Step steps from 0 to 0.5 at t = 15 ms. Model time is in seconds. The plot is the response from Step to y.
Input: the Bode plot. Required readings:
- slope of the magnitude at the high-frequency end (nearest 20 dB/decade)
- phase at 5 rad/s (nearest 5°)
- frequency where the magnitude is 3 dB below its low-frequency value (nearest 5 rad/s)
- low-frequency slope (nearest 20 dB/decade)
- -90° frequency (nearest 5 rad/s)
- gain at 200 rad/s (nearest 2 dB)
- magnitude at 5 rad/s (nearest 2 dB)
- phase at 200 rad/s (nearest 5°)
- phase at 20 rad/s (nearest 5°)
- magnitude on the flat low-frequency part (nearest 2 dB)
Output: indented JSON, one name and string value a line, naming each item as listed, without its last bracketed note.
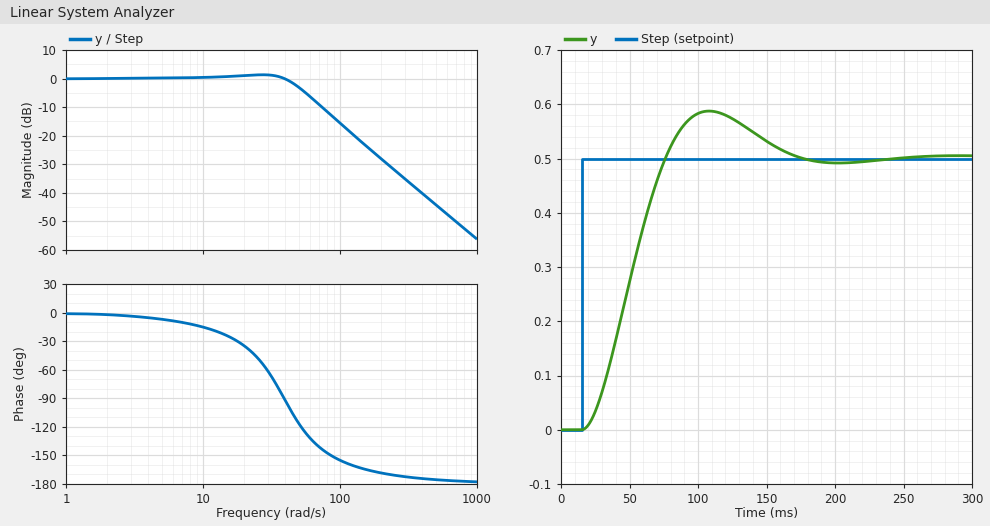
{
  "slope of the magnitude at the high-frequency end": "-40 dB/decade",
  "phase at 5 rad/s": "-5°",
  "frequency where the magnitude is 3 dB below its low-frequency value": "50 rad/s",
  "low-frequency slope": "0 dB/decade",
  "-90° frequency": "40 rad/s",
  "gain at 200 rad/s": "-28 dB",
  "magnitude at 5 rad/s": "0 dB",
  "phase at 200 rad/s": "-170°",
  "phase at 20 rad/s": "-35°",
  "magnitude on the flat low-frequency part": "0 dB"
}
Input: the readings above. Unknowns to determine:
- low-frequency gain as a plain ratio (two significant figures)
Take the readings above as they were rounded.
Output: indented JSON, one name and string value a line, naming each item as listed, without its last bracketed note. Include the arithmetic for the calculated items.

{
  "low-frequency gain as a plain ratio": "10^(0 / 20) = 1.0"
}
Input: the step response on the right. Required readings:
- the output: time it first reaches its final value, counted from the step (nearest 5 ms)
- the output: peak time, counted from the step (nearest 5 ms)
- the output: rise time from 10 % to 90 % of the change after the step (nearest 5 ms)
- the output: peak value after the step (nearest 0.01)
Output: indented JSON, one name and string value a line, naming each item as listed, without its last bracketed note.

{
  "the output: time it first reaches its final value, counted from the step": "60 ms",
  "the output: peak time, counted from the step": "95 ms",
  "the output: rise time from 10 % to 90 % of the change after the step": "40 ms",
  "the output: peak value after the step": "0.59"
}
